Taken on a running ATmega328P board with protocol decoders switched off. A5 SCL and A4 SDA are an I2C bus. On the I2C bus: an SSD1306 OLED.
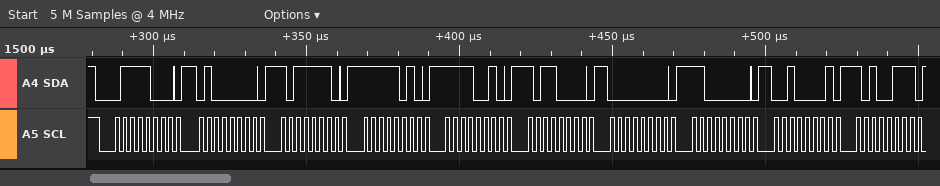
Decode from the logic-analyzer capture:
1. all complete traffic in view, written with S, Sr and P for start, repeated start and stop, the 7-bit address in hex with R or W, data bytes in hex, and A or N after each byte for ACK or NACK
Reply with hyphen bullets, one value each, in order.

- S 3CW A 40 A BE A FA A F2 A B0 A 00 A C0 A 21 A A7 A
